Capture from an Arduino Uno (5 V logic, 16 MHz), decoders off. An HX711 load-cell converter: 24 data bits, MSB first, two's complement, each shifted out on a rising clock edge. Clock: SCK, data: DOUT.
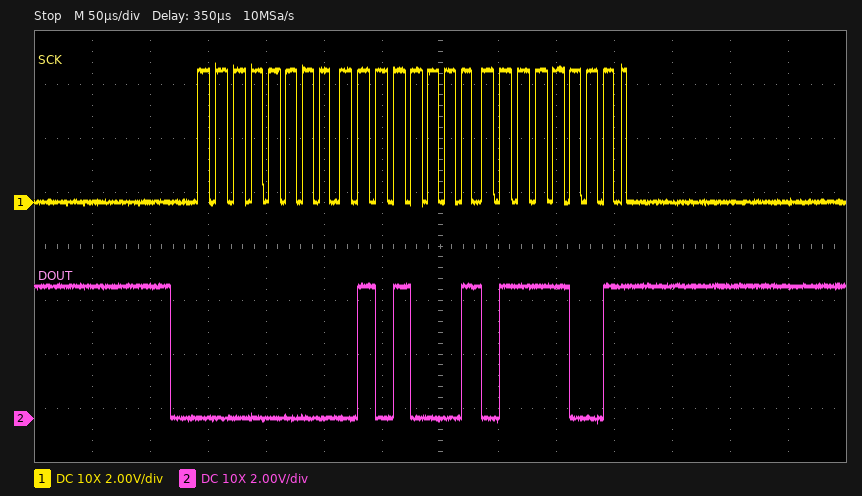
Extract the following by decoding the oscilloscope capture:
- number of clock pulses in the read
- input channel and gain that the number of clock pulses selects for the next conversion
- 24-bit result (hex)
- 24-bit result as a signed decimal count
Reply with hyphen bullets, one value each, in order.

- 25
- channel A, gain 128
- 0x005179
- 20857
